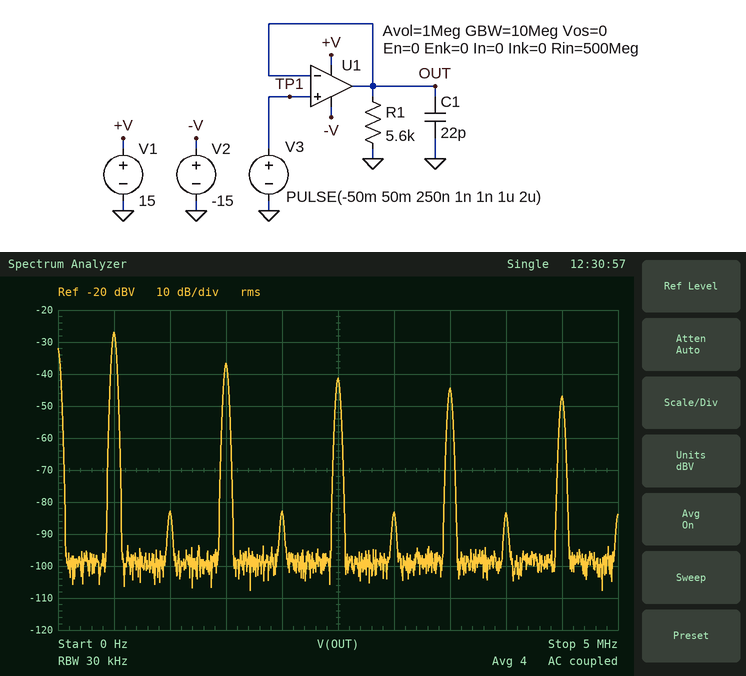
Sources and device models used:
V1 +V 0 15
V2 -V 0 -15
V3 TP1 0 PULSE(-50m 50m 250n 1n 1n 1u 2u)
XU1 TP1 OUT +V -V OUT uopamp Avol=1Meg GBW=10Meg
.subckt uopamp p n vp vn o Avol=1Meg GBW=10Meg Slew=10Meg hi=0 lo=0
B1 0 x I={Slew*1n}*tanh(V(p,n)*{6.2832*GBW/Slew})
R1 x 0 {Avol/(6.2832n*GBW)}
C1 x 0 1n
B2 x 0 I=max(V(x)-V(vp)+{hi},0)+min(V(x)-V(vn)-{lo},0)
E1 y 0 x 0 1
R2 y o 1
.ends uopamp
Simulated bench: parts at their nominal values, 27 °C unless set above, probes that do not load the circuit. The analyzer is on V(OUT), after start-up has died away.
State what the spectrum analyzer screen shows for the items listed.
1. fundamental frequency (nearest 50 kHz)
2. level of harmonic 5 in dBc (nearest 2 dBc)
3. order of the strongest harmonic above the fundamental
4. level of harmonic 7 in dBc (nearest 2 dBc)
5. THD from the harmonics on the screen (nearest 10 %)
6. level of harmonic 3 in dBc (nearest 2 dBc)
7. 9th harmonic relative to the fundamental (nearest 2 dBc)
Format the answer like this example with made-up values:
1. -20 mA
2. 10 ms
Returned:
1. 500 kHz
2. -14 dBc
3. 3
4. -18 dBc
5. 40 %
6. -10 dBc
7. -20 dBc
